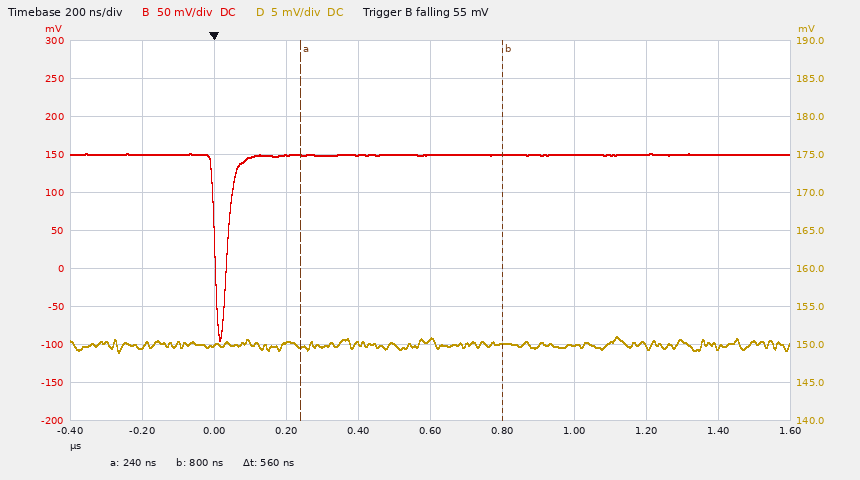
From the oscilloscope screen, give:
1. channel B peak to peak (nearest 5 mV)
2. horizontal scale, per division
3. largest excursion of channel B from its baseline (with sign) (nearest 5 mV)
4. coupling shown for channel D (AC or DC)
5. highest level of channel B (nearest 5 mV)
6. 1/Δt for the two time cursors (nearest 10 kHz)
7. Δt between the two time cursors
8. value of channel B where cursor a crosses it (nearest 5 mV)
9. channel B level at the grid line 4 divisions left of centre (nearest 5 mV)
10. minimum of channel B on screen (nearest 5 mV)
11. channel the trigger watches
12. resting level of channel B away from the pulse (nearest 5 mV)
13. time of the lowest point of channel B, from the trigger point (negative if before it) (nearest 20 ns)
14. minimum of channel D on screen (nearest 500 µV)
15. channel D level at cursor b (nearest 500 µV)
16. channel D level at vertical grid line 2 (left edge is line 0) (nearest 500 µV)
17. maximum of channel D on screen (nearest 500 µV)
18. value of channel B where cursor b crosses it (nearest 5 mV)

245 mV
200 ns
-245 mV
DC
150 mV
1.79 MHz
560 ns
150 mV
150 mV
-95 mV
channel B
150 mV
+20 ns
149.0 mV
150.0 mV
150.0 mV
151.0 mV
150 mV
